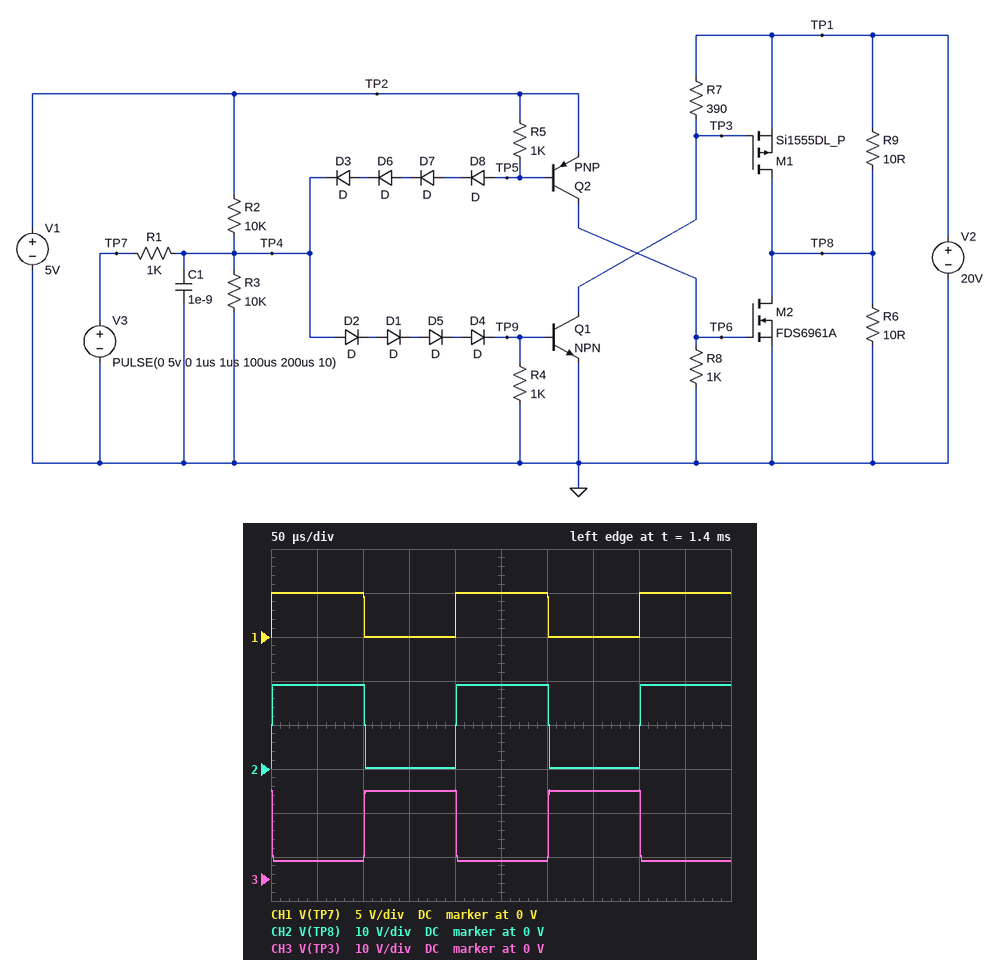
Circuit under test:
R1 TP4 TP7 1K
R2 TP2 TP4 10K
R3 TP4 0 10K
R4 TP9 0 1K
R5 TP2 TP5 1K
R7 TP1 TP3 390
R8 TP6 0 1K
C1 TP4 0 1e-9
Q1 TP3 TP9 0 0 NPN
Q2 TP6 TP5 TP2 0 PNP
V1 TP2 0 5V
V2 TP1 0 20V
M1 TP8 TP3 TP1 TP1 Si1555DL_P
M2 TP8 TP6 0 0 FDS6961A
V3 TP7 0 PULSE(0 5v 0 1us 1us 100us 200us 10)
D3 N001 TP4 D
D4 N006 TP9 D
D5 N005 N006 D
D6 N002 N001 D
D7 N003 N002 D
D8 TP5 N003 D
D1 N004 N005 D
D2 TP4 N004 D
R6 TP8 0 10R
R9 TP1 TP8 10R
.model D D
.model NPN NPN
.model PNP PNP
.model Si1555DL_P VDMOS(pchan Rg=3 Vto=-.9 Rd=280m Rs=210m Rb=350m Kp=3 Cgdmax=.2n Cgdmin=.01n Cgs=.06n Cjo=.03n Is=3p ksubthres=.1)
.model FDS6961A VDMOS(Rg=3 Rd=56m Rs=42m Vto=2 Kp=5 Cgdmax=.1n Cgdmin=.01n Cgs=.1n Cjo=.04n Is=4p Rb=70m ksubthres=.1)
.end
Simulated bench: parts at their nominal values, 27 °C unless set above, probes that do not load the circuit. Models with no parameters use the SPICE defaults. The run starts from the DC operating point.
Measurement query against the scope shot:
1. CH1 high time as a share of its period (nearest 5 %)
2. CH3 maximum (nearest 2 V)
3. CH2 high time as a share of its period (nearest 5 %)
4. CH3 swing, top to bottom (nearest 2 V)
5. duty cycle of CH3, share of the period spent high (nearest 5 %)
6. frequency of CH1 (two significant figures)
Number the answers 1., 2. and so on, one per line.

1. 50 %
2. 20 V
3. 50 %
4. 16 V
5. 50 %
6. 5.0 kHz
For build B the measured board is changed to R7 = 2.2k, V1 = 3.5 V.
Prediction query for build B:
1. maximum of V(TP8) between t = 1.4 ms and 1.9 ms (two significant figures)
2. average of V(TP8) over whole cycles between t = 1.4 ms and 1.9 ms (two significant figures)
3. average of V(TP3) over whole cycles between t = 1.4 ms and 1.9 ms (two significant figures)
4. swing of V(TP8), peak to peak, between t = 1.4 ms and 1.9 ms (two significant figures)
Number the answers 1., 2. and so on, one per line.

1. 19 V
2. 15 V
3. 10 V
4. 9.1 V
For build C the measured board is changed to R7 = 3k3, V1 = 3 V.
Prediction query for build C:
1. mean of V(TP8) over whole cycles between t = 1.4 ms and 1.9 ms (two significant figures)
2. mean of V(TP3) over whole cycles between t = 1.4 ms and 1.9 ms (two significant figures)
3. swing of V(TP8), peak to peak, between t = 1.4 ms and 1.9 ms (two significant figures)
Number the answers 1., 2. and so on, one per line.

1. 15 V
2. 10 V
3. 9.1 V
